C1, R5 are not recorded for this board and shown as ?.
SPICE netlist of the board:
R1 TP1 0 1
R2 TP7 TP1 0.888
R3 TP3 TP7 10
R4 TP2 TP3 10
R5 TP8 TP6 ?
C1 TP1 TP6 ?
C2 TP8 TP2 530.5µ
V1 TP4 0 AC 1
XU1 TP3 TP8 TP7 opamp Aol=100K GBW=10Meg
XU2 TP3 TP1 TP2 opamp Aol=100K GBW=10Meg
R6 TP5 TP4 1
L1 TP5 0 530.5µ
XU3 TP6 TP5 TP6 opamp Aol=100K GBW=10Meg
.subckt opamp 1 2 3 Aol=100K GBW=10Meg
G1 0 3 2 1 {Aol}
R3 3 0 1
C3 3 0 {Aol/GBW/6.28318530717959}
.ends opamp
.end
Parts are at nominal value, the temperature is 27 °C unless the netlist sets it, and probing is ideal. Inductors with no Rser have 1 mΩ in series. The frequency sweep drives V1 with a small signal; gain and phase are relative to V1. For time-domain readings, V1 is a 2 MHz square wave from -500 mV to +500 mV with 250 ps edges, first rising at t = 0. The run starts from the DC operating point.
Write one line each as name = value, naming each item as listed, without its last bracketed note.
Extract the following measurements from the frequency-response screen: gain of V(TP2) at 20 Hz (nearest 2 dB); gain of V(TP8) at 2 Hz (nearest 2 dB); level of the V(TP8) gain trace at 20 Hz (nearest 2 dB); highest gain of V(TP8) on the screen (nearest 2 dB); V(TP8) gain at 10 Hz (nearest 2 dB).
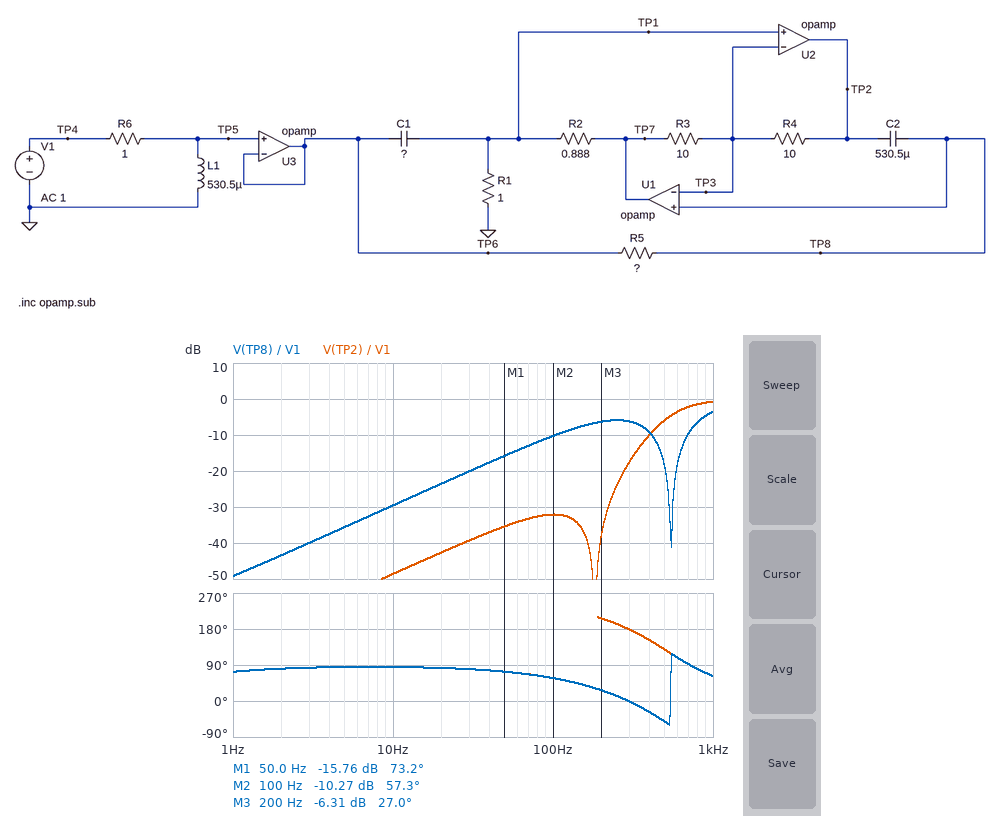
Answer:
gain of V(TP2) at 20 Hz = -42 dB
gain of V(TP8) at 2 Hz = -44 dB
level of the V(TP8) gain trace at 20 Hz = -24 dB
highest gain of V(TP8) on the screen = -4 dB
V(TP8) gain at 10 Hz = -30 dB
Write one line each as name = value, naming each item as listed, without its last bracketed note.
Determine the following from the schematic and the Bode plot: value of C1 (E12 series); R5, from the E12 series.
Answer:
value of C1 = 220 µF
R5, from the E12 series = 0.82 Ω
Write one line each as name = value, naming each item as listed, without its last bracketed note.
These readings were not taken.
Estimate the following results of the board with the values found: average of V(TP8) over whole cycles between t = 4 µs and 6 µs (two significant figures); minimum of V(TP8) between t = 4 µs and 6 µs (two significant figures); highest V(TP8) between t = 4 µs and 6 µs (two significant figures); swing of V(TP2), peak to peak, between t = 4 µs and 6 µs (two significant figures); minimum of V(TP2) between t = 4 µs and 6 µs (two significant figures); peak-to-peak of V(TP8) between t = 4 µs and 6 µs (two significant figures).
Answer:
average of V(TP8) over whole cycles between t = 4 µs and 6 µs = 480 mV
minimum of V(TP8) between t = 4 µs and 6 µs = -160 mV
highest V(TP8) between t = 4 µs and 6 µs = 1.1 V
swing of V(TP2), peak to peak, between t = 4 µs and 6 µs = 1.3 V
minimum of V(TP2) between t = 4 µs and 6 µs = -160 mV
peak-to-peak of V(TP8) between t = 4 µs and 6 µs = 1.3 V
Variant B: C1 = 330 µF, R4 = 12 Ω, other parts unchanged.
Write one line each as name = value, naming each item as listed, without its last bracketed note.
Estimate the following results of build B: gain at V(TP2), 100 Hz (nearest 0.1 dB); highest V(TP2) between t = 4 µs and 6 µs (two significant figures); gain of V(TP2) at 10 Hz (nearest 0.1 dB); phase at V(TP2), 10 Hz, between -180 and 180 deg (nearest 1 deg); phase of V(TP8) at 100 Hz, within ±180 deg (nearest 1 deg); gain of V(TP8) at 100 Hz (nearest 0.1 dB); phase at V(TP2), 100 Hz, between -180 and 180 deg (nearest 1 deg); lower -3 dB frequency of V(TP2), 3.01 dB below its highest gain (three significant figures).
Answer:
gain at V(TP2), 100 Hz = -27.9 dB
highest V(TP2) between t = 4 µs and 6 µs = 1.1 V
gain of V(TP2) at 10 Hz = -53.1 dB
phase at V(TP2), 10 Hz, between -180 and 180 deg = -95 deg
phase of V(TP8) at 100 Hz, within ±180 deg = 54 deg
gain of V(TP8) at 100 Hz = -10.4 dB
phase at V(TP2), 100 Hz, between -180 and 180 deg = -126 deg
lower -3 dB frequency of V(TP2), 3.01 dB below its highest gain = 401 Hz
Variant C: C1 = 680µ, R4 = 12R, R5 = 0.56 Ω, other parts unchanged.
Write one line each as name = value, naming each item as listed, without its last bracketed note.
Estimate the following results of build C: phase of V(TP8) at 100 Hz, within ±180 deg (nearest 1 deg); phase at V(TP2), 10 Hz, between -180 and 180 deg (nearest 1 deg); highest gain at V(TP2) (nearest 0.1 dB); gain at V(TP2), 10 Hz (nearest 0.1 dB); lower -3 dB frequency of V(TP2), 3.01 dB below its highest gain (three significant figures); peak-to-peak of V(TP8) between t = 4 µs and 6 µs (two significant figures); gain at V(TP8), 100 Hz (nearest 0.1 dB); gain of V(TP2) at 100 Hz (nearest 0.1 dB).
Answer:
phase of V(TP8) at 100 Hz, within ±180 deg = 59 deg
phase at V(TP2), 10 Hz, between -180 and 180 deg = -95 deg
highest gain at V(TP2) = 2.3 dB
gain at V(TP2), 10 Hz = -53.1 dB
lower -3 dB frequency of V(TP2), 3.01 dB below its highest gain = 301 Hz
peak-to-peak of V(TP8) between t = 4 µs and 6 µs = 1.3 V
gain at V(TP8), 100 Hz = -10.2 dB
gain of V(TP2) at 100 Hz = -25.9 dB
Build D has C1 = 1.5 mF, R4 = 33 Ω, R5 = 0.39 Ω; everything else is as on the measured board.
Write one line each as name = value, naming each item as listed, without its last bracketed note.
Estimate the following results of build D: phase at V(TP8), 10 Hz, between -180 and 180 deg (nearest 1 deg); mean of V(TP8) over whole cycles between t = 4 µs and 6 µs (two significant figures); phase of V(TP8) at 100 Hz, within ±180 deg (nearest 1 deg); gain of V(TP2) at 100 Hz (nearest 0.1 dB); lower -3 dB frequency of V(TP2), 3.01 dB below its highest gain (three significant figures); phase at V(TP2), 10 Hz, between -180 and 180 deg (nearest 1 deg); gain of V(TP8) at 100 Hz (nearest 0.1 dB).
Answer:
phase at V(TP8), 10 Hz, between -180 and 180 deg = 84 deg
mean of V(TP8) over whole cycles between t = 4 µs and 6 µs = 490 mV
phase of V(TP8) at 100 Hz, within ±180 deg = 41 deg
gain of V(TP2) at 100 Hz = -0.3 dB
lower -3 dB frequency of V(TP2), 3.01 dB below its highest gain = 130 Hz
phase at V(TP2), 10 Hz, between -180 and 180 deg = -96 deg
gain of V(TP8) at 100 Hz = -11.3 dB
